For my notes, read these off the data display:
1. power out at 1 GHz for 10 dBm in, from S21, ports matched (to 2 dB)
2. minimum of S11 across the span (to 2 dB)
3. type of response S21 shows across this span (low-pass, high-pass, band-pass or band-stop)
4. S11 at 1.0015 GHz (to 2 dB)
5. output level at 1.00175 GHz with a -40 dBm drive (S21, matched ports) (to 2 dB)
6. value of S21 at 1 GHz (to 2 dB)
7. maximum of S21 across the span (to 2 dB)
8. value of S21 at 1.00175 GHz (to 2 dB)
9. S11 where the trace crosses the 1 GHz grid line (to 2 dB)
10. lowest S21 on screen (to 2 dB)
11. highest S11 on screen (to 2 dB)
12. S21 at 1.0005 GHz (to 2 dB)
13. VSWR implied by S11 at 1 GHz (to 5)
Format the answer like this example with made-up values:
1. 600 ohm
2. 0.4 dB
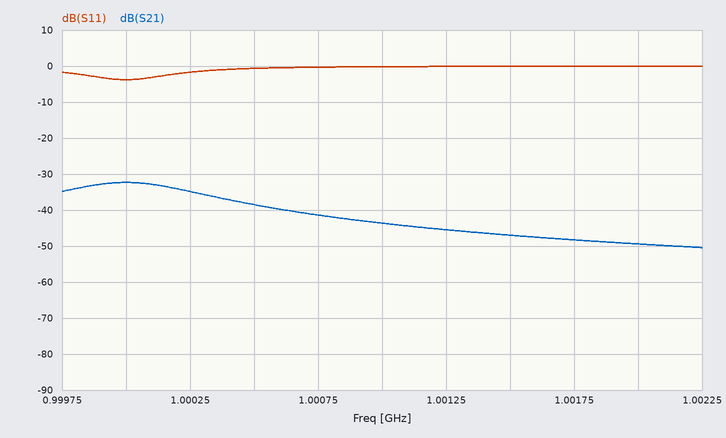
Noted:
1. -22 dBm
2. -4 dB
3. low-pass
4. 0 dB
5. -88 dBm
6. -32 dB
7. -32 dB
8. -48 dB
9. -4 dB
10. -50 dB
11. 0 dB
12. -38 dB
13. 5
